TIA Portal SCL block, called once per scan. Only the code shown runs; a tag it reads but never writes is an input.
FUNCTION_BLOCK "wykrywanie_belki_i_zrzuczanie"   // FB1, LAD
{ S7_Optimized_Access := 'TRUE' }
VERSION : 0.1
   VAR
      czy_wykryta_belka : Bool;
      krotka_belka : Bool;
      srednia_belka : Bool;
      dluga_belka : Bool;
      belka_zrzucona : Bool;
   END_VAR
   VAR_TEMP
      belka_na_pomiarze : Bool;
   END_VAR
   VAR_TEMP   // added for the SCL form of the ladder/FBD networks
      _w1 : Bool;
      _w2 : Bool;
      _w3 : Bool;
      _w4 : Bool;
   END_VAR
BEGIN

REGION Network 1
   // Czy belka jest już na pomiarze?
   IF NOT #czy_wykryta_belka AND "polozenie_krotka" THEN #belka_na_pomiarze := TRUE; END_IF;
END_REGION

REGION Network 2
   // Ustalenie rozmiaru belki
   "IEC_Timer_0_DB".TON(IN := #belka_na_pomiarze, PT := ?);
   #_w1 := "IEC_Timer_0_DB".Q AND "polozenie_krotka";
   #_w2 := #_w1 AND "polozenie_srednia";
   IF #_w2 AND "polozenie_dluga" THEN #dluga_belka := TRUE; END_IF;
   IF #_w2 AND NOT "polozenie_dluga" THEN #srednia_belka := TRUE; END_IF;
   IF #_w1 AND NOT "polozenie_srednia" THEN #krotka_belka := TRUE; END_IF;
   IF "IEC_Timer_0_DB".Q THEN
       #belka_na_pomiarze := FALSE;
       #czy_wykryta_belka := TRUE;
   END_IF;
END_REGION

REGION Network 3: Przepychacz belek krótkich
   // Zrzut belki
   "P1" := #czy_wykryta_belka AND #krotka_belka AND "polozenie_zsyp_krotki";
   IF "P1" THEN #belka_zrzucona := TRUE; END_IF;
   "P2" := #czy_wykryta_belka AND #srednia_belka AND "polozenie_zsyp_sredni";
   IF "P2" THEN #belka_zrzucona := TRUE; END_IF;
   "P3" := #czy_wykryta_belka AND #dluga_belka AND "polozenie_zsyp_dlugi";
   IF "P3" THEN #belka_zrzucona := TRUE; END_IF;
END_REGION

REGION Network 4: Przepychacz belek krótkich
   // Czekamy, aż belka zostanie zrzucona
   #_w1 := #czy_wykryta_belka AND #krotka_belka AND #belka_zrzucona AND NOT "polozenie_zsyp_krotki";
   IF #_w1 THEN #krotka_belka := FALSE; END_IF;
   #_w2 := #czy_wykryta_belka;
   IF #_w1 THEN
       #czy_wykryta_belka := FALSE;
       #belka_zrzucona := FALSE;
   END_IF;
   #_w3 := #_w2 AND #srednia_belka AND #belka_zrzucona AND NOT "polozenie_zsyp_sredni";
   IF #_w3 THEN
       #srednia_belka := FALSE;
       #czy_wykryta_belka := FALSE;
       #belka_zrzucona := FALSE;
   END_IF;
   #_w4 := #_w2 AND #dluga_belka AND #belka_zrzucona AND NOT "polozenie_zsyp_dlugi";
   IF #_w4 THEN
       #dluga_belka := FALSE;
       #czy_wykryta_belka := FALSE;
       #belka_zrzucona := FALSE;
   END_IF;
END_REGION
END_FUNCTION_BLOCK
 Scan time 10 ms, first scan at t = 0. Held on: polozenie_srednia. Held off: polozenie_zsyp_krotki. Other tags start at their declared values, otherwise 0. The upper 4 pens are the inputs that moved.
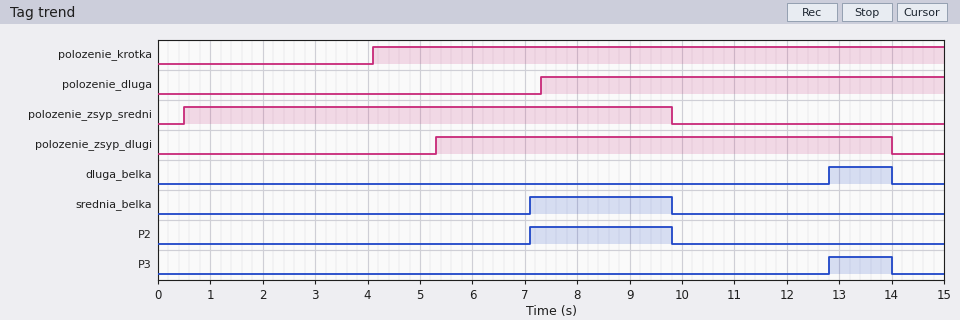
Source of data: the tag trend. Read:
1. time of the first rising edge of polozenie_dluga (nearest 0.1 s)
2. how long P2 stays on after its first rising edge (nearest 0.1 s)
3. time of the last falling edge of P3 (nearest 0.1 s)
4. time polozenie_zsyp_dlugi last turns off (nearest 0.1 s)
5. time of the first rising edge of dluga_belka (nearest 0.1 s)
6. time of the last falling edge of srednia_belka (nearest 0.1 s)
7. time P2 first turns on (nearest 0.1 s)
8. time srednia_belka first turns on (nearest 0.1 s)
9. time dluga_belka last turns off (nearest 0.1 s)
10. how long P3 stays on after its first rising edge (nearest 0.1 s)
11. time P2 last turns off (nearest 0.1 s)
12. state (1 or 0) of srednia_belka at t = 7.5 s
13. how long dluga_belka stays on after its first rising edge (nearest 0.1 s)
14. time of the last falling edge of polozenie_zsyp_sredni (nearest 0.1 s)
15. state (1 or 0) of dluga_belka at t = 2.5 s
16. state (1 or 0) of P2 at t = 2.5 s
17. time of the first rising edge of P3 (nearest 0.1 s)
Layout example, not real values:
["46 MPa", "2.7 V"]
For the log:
["7.3 s", "2.7 s", "14.0 s", "14.0 s", "12.8 s", "9.8 s", "7.1 s", "7.1 s", "14.0 s", "1.2 s", "9.8 s", "1", "1.2 s", "9.8 s", "0", "0", "12.8 s"]
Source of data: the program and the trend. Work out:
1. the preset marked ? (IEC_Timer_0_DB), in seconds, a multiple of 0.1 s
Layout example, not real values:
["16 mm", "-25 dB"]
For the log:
["3.0 s"]
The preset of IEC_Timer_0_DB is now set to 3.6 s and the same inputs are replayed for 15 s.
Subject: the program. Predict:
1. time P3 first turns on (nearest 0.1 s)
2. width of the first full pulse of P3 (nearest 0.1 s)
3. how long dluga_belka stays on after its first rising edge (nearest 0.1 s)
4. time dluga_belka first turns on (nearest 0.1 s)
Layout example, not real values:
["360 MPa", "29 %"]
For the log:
["7.7 s", "6.3 s", "6.3 s", "7.7 s"]
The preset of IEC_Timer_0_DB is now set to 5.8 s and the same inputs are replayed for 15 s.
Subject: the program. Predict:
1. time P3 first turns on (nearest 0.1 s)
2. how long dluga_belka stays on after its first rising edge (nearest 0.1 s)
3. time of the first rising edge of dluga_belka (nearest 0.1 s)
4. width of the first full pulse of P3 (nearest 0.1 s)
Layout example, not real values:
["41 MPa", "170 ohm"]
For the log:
["9.9 s", "4.1 s", "9.9 s", "4.1 s"]
